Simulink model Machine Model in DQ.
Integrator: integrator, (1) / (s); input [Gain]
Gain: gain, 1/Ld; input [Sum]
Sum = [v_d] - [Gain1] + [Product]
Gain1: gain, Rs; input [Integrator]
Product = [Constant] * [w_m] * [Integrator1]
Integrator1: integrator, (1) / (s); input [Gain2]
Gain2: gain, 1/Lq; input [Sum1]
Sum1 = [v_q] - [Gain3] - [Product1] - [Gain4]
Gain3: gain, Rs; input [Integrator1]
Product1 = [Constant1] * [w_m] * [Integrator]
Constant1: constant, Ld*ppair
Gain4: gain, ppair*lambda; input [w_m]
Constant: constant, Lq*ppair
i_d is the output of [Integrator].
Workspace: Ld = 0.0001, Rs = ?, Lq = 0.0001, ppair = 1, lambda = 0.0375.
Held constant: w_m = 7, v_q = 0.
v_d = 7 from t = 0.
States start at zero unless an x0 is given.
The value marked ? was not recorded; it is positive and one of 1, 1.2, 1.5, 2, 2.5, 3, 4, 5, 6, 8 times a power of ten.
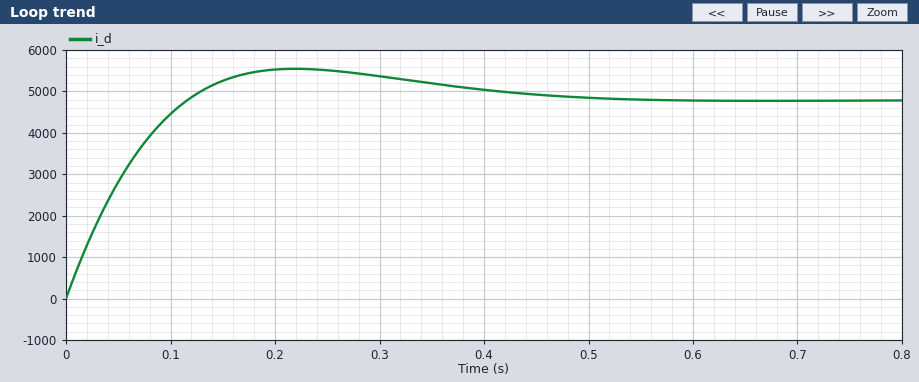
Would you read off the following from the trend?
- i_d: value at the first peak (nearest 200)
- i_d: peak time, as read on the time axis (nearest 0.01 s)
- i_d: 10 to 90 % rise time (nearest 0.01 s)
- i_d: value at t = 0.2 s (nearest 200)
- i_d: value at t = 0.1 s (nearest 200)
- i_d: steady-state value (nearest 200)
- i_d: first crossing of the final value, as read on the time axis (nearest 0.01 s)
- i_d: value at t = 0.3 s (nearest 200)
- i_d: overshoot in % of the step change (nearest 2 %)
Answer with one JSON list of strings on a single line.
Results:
["5600", "0.22 s", "0.09 s", "5600", "4400", "4800", "0.12 s", "5400", "16 %"]
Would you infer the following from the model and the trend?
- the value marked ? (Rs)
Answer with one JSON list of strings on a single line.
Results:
["0.0008"]
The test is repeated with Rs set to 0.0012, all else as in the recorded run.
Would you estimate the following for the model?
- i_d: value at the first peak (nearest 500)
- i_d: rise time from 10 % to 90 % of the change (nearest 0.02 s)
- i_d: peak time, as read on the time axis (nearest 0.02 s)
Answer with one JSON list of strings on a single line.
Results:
["4500", "0.10 s", "0.22 s"]
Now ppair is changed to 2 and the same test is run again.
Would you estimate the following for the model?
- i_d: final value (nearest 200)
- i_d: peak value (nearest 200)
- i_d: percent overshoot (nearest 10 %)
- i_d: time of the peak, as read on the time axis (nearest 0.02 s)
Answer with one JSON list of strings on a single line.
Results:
["1800", "3400", "90 %", "0.10 s"]
